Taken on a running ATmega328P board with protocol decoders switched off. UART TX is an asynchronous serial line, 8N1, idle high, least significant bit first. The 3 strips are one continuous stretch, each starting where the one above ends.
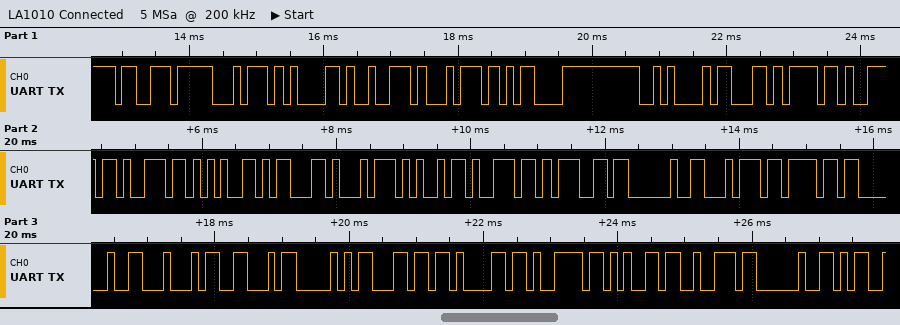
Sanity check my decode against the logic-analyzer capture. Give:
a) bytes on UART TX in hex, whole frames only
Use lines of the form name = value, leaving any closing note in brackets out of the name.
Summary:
bytes on UART TX in hex, whole frames only = 73 74 61 72 74 0D 0A 63 6F 6E 6E 65 63 74 69 6E 67 20 74 6F 20 44 46 50 6C 61 79 65 72 20
